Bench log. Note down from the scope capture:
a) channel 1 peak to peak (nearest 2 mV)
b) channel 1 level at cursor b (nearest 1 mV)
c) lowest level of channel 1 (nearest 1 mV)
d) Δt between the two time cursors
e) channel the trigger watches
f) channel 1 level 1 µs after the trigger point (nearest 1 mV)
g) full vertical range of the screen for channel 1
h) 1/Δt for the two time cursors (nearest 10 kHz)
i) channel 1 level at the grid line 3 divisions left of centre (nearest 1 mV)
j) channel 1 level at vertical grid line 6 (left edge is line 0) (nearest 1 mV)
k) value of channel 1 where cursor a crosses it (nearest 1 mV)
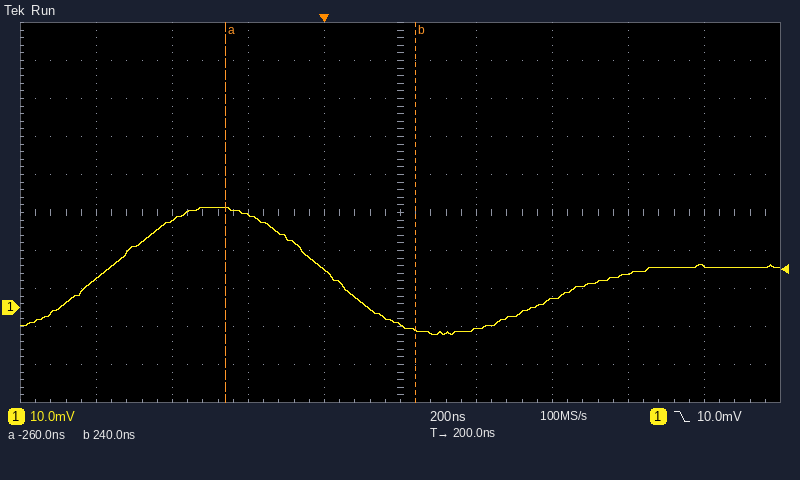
34 mV
-6 mV
-7 mV
500 ns
channel 1
11 mV
100 mV
2.00 MHz
23 mV
-6 mV
26 mV
